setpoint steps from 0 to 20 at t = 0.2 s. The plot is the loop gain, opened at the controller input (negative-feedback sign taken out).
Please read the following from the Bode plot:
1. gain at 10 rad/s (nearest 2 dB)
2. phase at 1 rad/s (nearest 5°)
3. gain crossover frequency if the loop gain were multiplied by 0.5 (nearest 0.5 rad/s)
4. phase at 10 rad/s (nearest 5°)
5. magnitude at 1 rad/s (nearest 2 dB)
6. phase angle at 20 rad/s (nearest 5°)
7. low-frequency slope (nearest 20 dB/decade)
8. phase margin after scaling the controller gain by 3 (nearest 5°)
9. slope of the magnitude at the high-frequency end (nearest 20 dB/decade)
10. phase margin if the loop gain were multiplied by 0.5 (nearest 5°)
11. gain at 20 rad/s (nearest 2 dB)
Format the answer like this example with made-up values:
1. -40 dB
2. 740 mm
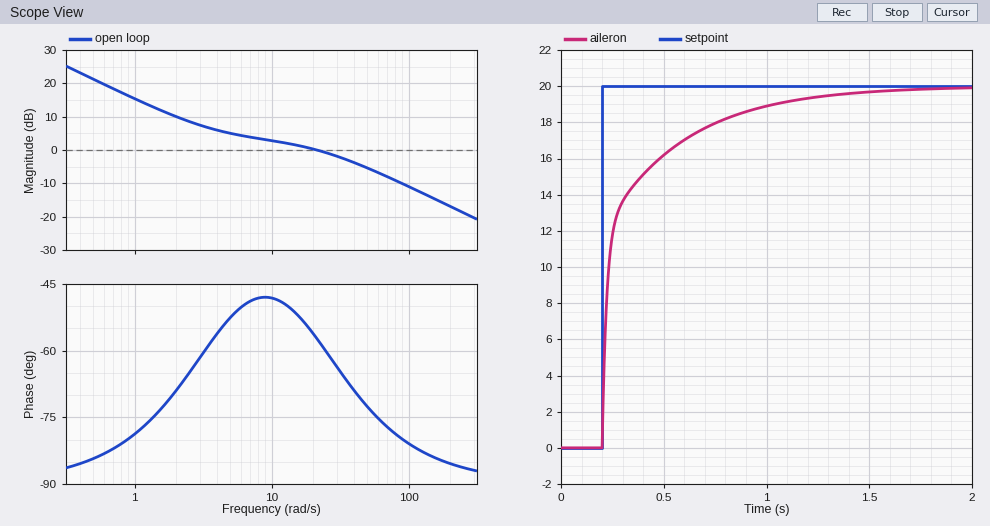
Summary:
1. 2 dB
2. -80°
3. 4.0 rad/s
4. -50°
5. 16 dB
6. -55°
7. -20 dB/decade
8. 100°
9. -20 dB/decade
10. 125°
11. 0 dB
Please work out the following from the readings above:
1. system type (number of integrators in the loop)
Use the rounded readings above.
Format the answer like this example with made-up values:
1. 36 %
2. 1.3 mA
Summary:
1. 1
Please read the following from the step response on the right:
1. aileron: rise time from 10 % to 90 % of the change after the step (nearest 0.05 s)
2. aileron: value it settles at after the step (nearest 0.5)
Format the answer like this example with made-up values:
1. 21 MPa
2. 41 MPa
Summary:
1. 0.55 s
2. 20.0
